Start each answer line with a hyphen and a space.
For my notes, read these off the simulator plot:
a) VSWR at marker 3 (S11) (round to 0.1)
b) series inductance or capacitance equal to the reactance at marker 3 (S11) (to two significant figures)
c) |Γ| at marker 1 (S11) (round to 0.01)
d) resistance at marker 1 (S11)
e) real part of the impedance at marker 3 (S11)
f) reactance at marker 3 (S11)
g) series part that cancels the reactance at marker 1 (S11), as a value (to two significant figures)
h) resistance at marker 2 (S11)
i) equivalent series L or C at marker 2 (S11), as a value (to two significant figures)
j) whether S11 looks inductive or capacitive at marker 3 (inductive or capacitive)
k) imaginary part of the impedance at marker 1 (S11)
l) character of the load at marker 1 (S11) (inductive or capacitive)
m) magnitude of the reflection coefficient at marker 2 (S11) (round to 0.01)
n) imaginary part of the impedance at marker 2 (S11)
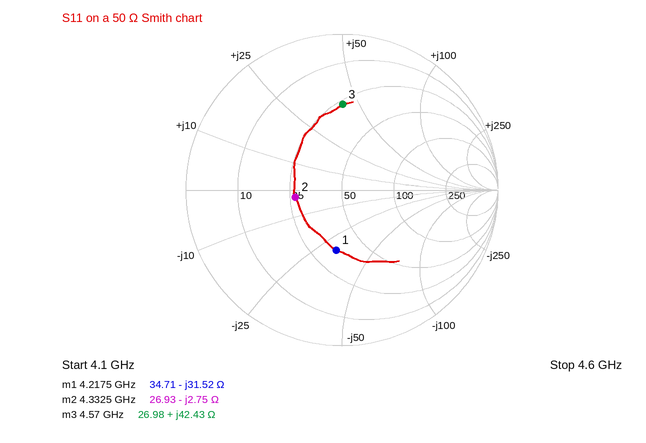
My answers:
- 3.4
- 1.5 nH
- 0.39
- 34.71 Ω
- 26.98 Ω
- +42.43 Ω
- 1.2 nH
- 26.93 Ω
- 13 pF
- inductive
- -31.52 Ω
- capacitive
- 0.30
- -2.75 Ω
